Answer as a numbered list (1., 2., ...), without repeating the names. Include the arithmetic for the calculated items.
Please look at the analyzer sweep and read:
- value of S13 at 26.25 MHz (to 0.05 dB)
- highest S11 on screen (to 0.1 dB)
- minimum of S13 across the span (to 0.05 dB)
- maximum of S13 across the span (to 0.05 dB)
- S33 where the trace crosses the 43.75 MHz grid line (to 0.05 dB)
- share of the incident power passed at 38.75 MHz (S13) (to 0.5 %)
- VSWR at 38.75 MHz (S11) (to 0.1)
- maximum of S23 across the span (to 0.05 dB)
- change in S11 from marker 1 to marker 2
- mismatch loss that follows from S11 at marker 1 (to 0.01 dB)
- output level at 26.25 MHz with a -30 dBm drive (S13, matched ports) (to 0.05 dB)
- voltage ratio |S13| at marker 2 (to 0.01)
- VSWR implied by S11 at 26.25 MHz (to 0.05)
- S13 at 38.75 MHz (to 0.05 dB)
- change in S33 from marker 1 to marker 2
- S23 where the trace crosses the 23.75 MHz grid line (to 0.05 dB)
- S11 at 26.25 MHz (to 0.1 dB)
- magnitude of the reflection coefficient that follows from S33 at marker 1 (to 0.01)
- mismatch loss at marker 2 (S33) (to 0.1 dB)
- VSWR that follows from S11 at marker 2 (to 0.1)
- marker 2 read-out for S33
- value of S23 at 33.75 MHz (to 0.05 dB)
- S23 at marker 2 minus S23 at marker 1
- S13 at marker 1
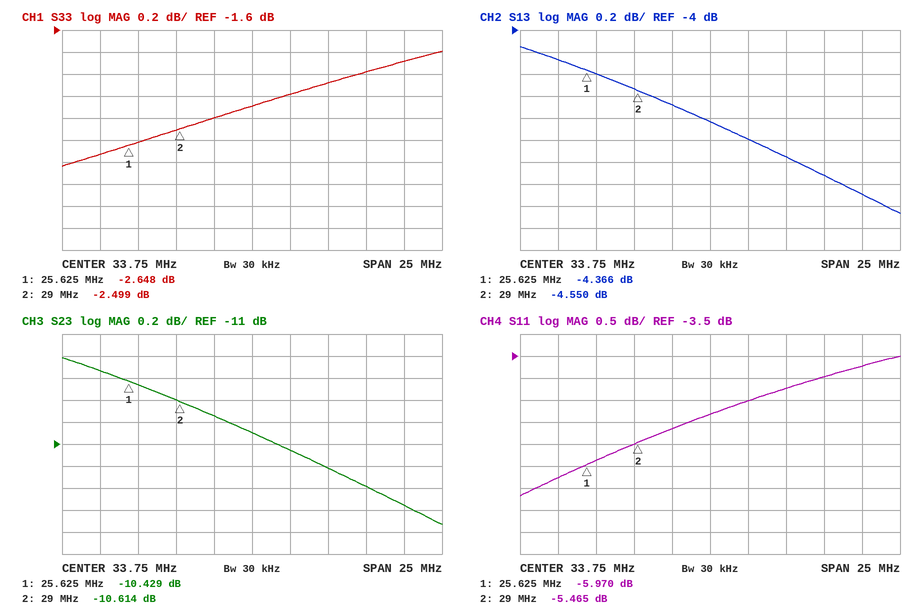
1. -4.40 dB
2. -3.5 dB
3. -5.65 dB
4. -4.15 dB
5. -1.90 dB
6. 10^(-5.15/10) ≈ 30.5 %
7. |Γ| = 10^(-4.2/20) = 0.6166; VSWR = (1 + 0.6166)/(1 − 0.6166) ≈ 4.2
8. -10.20 dB
9. -5.465 − (-5.97) = 0.505 dB
10. −10 log10(1 − 10^(-5.97/10)) ≈ 1.27 dB
11. -30 dBm + (-4.40 dB) = -34.40 dBm
12. 10^(-4.55/20) ≈ 0.59
13. |Γ| = 10^(-5.9/20) = 0.5070; VSWR = (1 + 0.5070)/(1 − 0.5070) ≈ 3.06, so 3.05 to the nearest 0.05
14. -5.15 dB
15. -2.499 − (-2.648) = 0.149 dB
16. -10.35 dB
17. -5.9 dB
18. 10^(-2.648/20) ≈ 0.74
19. −10 log10(1 − 10^(-2.499/10)) ≈ 3.6 dB
20. (1 + 0.5330)/(1 − 0.5330) ≈ 3.3
21. -2.499 dB
22. -10.90 dB
23. -10.614 − (-10.429) = -0.185 dB
24. -4.366 dB
